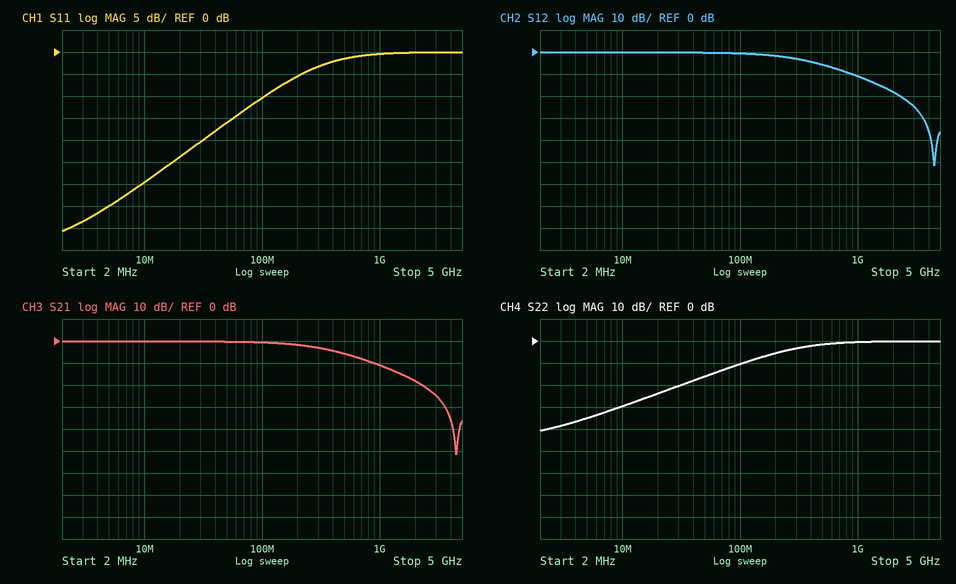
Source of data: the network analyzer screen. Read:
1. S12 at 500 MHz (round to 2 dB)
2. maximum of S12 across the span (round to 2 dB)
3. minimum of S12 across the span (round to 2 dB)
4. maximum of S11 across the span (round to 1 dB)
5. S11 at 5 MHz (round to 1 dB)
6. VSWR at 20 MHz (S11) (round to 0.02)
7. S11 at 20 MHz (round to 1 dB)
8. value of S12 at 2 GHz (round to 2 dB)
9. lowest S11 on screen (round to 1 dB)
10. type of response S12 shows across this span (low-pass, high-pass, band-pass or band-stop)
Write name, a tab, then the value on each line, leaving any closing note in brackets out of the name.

S12 at 500 MHz	-6 dB
maximum of S12 across the span	0 dB
minimum of S12 across the span	-52 dB
maximum of S11 across the span	0 dB
S11 at 5 MHz	-35 dB
VSWR at 20 MHz (S11)	1.14
S11 at 20 MHz	-24 dB
value of S12 at 2 GHz	-18 dB
lowest S11 on screen	-41 dB
type of response S12 shows across this span	low-pass
